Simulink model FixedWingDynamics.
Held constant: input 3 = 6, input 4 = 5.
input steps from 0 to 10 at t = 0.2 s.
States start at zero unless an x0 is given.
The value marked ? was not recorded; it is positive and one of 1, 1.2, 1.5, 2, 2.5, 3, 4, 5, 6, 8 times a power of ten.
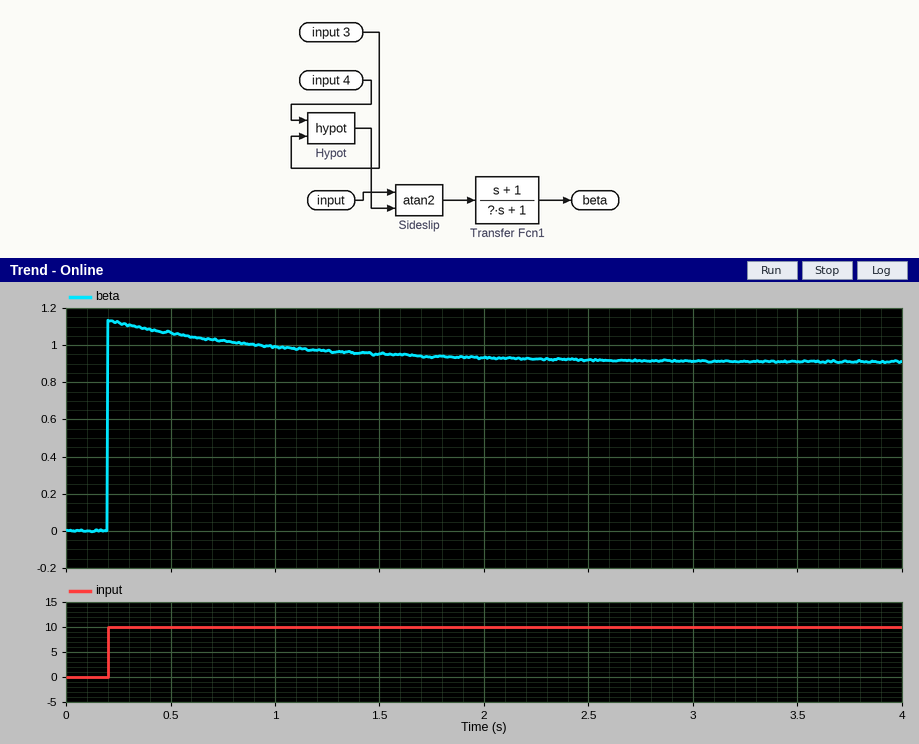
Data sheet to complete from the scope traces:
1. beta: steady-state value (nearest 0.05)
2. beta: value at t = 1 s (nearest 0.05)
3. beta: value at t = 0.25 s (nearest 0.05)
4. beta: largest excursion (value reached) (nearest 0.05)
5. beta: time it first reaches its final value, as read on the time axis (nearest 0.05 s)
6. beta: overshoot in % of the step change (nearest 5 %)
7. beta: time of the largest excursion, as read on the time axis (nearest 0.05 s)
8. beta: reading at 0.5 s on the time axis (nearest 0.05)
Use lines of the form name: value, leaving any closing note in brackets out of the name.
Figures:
beta: steady-state value: 0.90
beta: value at t = 1 s: 1.00
beta: value at t = 0.25 s: 1.10
beta: largest excursion (value reached): 1.15
beta: time it first reaches its final value, as read on the time axis: 0.20 s
beta: overshoot in % of the step change: 25 %
beta: time of the largest excursion, as read on the time axis: 0.20 s
beta: reading at 0.5 s on the time axis: 1.05
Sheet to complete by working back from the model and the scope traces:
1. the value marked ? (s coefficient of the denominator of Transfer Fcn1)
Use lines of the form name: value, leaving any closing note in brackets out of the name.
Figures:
the value marked ?: 0.8
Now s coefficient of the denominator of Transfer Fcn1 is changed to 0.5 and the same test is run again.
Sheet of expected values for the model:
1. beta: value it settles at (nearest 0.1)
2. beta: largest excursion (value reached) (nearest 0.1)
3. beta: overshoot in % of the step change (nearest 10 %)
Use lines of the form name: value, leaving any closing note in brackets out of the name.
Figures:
beta: value it settles at: 0.9
beta: largest excursion (value reached): 1.8
beta: overshoot in % of the step change: 100 %
